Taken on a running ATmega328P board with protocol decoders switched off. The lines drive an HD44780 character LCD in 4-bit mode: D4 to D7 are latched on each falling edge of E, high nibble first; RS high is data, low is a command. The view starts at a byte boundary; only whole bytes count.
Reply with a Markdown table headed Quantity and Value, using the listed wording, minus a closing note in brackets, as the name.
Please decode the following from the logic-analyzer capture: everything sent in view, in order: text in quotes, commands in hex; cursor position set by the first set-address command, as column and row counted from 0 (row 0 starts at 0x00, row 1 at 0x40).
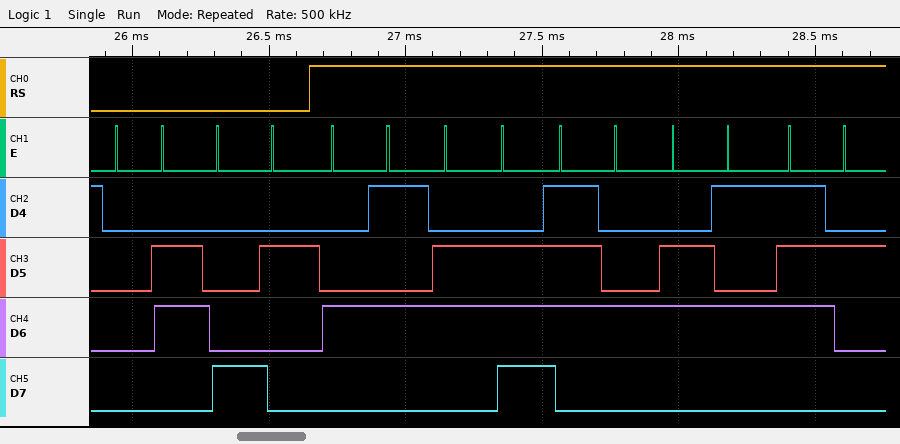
| Quantity | Value |
|---|---|
| everything sent in view, in order: text in quotes, commands in hex | 0x06 0x82 "Enter" |
| cursor position set by the first set-address command, as column and row counted from 0 | column 2, row 0 |
